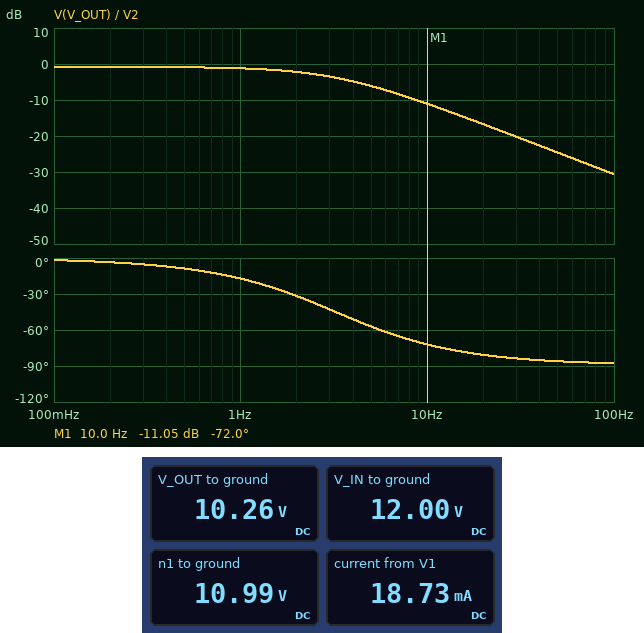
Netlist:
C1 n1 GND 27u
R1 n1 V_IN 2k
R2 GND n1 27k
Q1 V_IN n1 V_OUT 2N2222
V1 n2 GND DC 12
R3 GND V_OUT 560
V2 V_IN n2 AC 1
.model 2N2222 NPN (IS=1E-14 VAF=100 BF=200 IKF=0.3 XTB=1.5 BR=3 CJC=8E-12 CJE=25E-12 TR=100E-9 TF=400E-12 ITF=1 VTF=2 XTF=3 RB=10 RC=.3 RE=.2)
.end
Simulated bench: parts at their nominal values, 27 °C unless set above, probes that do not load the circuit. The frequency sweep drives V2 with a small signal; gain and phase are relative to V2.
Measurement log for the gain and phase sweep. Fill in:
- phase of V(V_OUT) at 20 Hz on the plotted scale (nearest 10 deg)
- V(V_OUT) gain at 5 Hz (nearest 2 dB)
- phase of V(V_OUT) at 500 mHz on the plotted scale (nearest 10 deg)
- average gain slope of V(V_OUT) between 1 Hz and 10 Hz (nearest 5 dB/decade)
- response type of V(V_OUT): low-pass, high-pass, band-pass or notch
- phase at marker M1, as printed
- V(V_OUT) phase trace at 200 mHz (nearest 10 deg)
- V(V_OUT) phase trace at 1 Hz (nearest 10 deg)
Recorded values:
-80 deg
-6 dB
-10 deg
-10 dB/decade
low-pass
-72.0 deg
0 deg
-20 deg
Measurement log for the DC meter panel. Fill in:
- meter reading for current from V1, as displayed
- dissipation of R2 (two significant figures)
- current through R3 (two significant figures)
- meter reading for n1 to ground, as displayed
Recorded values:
18.73 mA
4.5 mW
18 mA
10.99 V
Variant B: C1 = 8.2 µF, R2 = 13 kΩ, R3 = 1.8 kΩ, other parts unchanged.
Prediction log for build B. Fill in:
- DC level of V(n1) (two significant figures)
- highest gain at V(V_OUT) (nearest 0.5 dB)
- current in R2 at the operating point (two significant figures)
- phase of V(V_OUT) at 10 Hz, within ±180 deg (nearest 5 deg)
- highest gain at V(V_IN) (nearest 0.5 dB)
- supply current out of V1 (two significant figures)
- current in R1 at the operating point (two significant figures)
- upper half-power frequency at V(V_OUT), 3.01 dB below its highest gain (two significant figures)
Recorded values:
10 V
-1.5 dB
800 µA
-40 deg
0 dB
6.2 mA
820 µA
11 Hz
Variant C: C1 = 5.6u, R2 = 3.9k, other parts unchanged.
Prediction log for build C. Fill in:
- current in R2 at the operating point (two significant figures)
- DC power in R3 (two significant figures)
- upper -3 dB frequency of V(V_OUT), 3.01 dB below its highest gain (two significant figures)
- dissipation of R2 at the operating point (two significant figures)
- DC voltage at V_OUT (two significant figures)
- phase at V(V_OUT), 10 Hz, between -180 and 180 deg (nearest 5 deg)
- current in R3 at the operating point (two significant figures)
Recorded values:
2.0 mA
91 mW
22 Hz
16 mW
7.1 V
-25 deg
13 mA
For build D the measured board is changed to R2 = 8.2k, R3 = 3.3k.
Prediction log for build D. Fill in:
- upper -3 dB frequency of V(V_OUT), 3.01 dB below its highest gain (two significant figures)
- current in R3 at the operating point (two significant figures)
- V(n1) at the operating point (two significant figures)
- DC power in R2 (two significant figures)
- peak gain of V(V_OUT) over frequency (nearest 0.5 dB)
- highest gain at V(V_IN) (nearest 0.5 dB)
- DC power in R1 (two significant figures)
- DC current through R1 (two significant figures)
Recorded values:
3.7 Hz
2.7 mA
9.6 V
11 mW
-2.0 dB
0 dB
2.8 mW
1.2 mA
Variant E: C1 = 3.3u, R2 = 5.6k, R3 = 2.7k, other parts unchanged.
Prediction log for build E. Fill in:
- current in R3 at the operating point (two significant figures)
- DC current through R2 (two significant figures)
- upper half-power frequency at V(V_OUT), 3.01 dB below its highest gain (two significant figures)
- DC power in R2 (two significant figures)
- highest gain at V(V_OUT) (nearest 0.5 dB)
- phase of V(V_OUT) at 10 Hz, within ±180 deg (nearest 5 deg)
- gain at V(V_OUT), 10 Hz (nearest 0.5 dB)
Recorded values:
3.0 mA
1.6 mA
33 Hz
14 mW
-2.5 dB
-15 deg
-3.0 dB
